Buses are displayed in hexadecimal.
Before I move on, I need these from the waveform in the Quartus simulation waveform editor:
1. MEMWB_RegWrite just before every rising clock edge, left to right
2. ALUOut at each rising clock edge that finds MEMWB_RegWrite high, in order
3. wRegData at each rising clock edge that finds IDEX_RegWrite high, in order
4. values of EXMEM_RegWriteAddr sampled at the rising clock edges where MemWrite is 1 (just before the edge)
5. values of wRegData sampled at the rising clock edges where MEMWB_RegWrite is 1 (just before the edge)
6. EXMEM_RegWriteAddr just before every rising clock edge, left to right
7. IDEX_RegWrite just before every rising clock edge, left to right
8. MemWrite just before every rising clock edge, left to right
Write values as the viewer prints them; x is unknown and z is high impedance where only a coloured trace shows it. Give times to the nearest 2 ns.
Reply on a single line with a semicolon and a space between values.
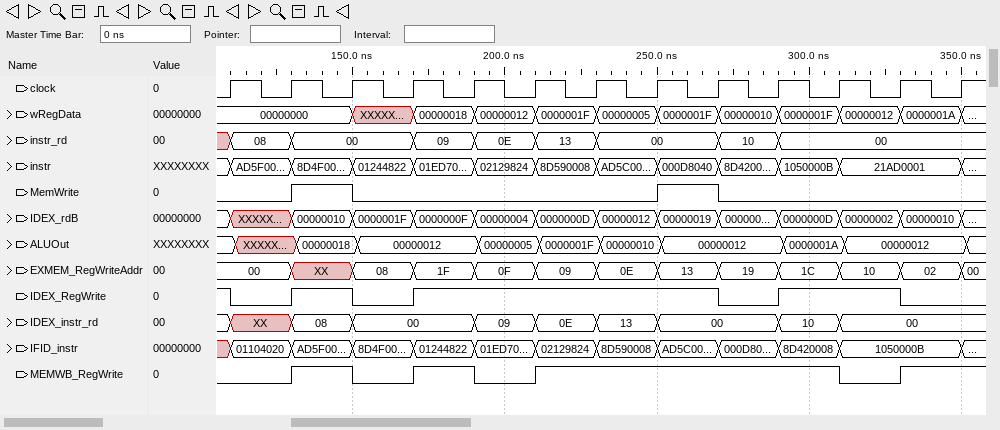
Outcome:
0 0 1 0 1 0 1 1 1 1 1 0 1; 00000018, 00000012, 0000001F, 00000010, 00000012, 00000012, 0000001A, 00000012; 00000000, 00000000, 00000018, 00000012, 0000001F, 00000005, 0000001F, 0000001F, 00000012; XX, 13; 00000000, 00000018, 0000001F, 00000005, 0000001F, 00000010, 0000001F, 0000001A; 00, 00, XX, 08, 1F, 0F, 09, 0E, 13, 19, 1C, 10, 02; 1 0 1 0 1 1 1 1 1 0 1 1 0; 0 0 1 0 0 0 0 0 1 0 0 0 0
